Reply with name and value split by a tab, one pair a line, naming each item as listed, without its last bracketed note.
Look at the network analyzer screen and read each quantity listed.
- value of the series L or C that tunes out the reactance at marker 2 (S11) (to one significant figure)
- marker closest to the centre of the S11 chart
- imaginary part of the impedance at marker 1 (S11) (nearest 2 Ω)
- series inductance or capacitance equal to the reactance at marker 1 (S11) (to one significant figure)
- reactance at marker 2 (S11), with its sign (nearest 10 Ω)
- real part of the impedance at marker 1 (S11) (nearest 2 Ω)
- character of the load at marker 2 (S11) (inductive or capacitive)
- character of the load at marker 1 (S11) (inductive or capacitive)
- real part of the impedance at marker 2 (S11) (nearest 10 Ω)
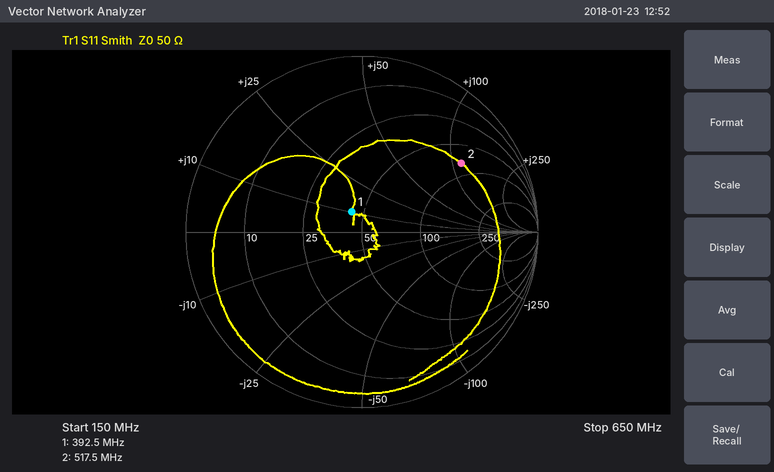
value of the series L or C that tunes out the reactance at marker 2 (S11)	3 pF
marker closest to the centre of the S11 chart	marker 1
imaginary part of the impedance at marker 1 (S11)	+10 Ω
series inductance or capacitance equal to the reactance at marker 1 (S11)	4 nH
reactance at marker 2 (S11), with its sign	+110 Ω
real part of the impedance at marker 1 (S11)	44 Ω
character of the load at marker 2 (S11)	inductive
character of the load at marker 1 (S11)	inductive
real part of the impedance at marker 2 (S11)	80 Ω
